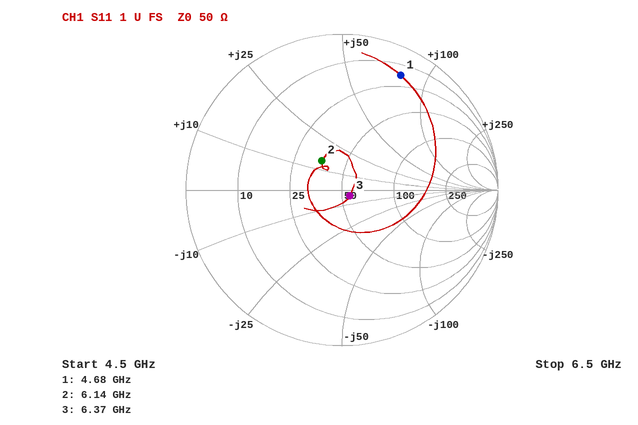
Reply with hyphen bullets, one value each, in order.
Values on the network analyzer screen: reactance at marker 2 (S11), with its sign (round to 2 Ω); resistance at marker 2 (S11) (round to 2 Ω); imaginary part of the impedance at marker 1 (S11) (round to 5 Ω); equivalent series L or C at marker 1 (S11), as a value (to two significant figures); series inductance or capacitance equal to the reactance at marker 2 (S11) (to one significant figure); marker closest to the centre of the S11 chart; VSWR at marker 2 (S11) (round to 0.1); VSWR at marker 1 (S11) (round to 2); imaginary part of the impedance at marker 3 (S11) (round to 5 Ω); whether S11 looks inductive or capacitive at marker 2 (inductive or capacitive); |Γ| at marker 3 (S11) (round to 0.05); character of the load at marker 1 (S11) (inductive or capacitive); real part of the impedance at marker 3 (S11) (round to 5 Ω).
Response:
- +14 Ω
- 36 Ω
- +80 Ω
- 2.7 nH
- 400 pH
- marker 3
- 1.6
- 10
- -5 Ω
- inductive
- 0.05
- inductive
- 55 Ω
